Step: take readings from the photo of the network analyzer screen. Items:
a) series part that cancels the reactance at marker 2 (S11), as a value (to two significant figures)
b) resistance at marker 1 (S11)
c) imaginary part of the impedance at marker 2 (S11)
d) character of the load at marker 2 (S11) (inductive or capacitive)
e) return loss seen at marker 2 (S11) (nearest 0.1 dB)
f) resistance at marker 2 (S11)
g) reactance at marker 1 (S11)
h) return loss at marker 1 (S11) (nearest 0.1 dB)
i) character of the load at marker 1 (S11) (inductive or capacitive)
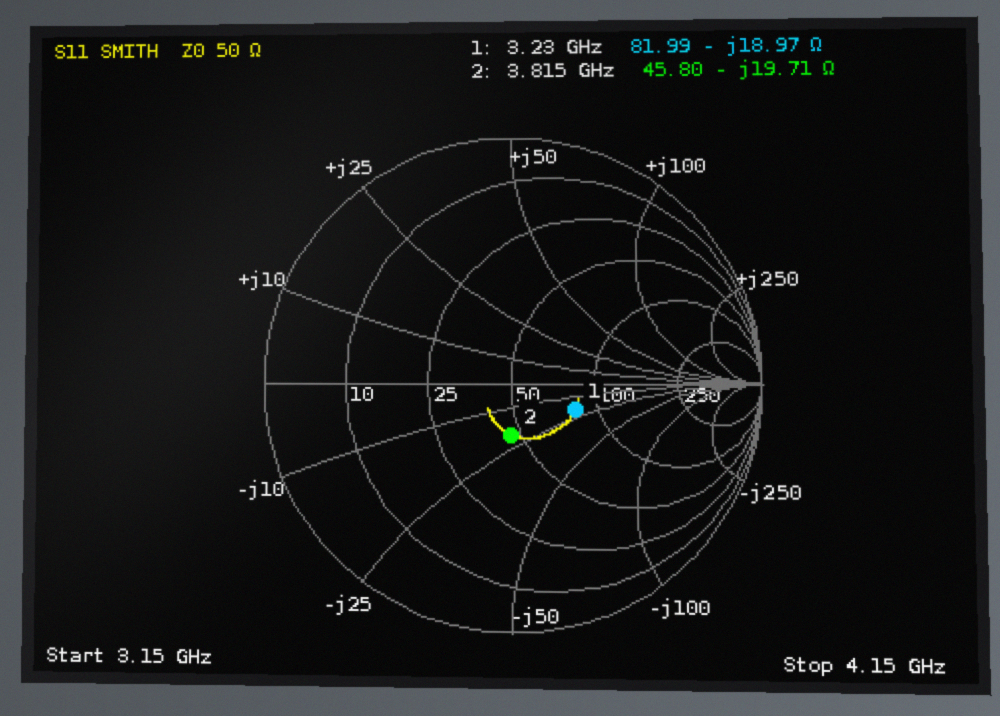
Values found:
820 pH
81.99 Ω
-19.71 Ω
capacitive
13.7 dB
45.80 Ω
-18.97 Ω
11.1 dB
capacitive
